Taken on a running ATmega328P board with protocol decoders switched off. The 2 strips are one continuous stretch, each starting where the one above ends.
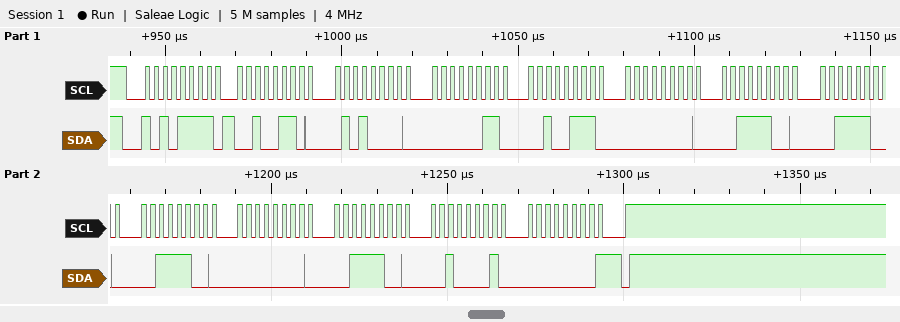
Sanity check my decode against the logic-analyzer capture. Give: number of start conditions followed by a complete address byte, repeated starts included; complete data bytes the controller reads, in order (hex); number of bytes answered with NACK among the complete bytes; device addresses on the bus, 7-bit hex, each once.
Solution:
1
26 50 03 27 00 3C 3C 3C 00 3C 21 00
1
0x57
